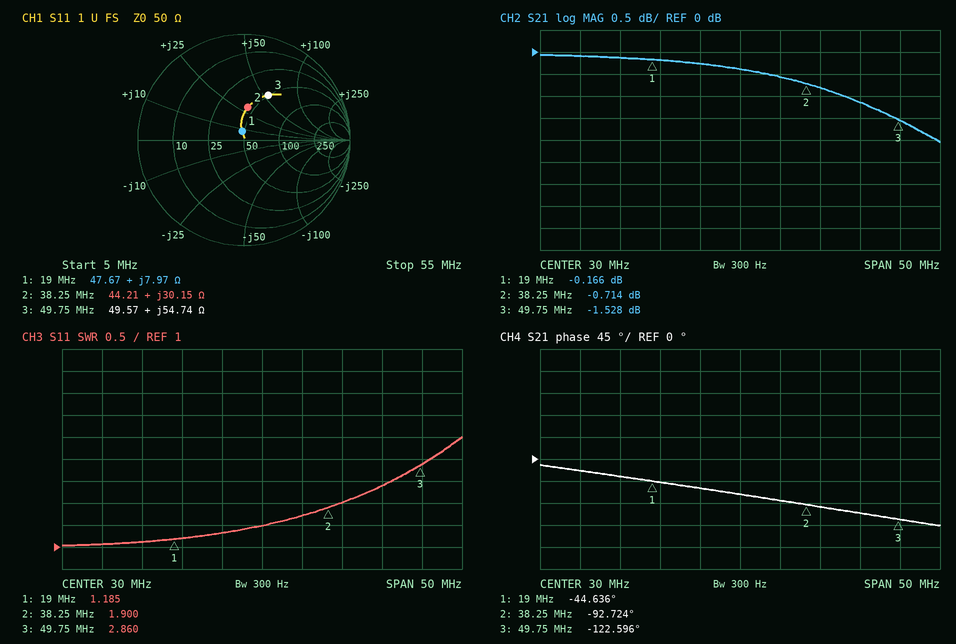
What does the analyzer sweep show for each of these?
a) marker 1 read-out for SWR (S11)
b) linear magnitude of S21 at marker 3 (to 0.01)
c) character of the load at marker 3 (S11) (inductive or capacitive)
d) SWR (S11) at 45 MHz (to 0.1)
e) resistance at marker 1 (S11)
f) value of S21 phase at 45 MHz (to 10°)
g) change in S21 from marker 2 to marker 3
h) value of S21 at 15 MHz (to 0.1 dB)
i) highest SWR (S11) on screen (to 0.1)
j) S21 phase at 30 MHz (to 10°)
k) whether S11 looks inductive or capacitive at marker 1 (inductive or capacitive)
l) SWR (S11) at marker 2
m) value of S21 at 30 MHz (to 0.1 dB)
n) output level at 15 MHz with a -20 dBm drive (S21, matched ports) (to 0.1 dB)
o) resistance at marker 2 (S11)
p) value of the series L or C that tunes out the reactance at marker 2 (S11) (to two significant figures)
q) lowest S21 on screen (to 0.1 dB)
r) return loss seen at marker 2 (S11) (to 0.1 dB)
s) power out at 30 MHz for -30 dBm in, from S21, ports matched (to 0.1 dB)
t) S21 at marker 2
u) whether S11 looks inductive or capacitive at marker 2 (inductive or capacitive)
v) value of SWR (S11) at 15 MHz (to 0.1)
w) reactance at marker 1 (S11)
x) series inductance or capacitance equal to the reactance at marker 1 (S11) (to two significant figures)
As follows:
1.185
0.84
inductive
2.4
47.67 Ω
-110°
-0.814 dB
-0.1 dB
3.5
-70°
inductive
1.900
-0.4 dB
-20.1 dBm
44.21 Ω
140 pF
-2.0 dB
10.2 dB
-30.4 dBm
-0.714 dB
inductive
1.1
+7.97 Ω
67 nH
